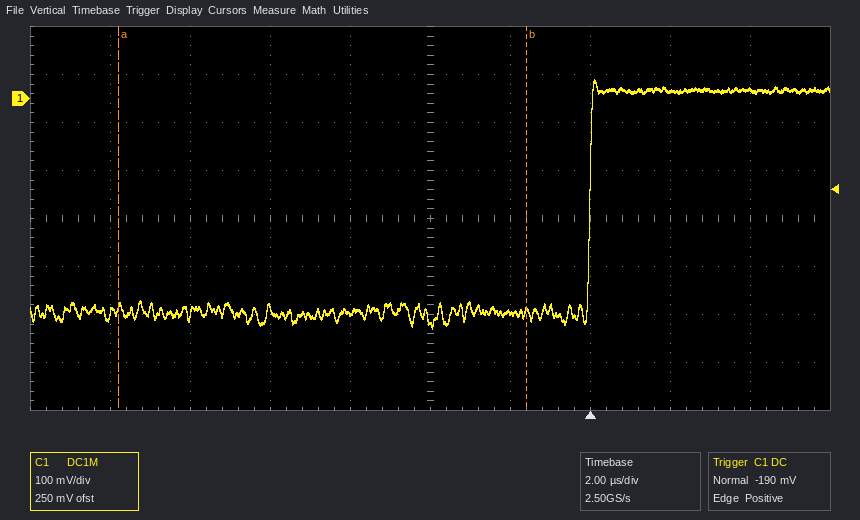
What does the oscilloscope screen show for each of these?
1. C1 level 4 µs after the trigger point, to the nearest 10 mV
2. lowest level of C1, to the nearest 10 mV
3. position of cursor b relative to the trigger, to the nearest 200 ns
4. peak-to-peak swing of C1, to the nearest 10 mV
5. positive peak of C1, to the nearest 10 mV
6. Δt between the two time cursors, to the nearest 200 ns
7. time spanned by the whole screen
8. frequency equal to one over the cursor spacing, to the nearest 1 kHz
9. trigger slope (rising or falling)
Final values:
20 mV
-480 mV
-1.6 µs
520 mV
40 mV
10.2 µs
20 µs
98 kHz
rising
